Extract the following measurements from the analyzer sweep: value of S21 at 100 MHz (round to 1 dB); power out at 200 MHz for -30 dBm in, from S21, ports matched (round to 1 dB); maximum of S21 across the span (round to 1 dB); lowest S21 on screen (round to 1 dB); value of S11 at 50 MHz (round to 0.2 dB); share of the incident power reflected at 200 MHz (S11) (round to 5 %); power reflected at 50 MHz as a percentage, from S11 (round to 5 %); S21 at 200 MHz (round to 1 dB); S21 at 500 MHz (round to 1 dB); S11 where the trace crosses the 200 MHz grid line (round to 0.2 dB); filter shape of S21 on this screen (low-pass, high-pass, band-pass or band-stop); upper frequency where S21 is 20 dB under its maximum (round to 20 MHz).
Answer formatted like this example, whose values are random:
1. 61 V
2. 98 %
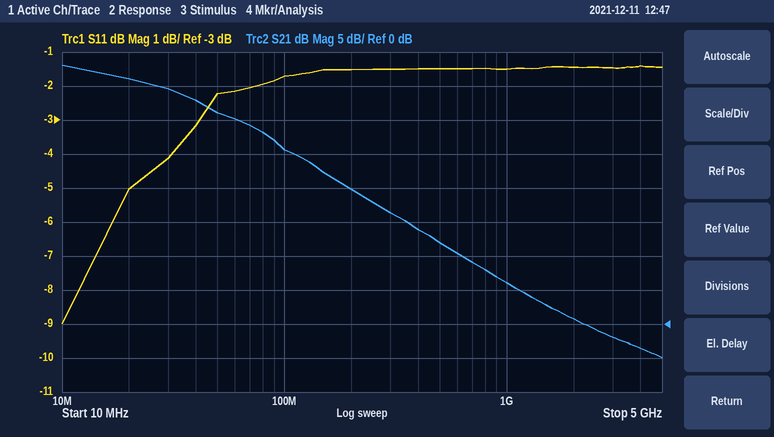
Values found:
1. 26 dB
2. -10 dBm
3. 38 dB
4. -5 dB
5. -2.2 dB
6. 70 %
7. 60 %
8. 20 dB
9. 12 dB
10. -1.6 dB
11. low-pass
12. 240 MHz
